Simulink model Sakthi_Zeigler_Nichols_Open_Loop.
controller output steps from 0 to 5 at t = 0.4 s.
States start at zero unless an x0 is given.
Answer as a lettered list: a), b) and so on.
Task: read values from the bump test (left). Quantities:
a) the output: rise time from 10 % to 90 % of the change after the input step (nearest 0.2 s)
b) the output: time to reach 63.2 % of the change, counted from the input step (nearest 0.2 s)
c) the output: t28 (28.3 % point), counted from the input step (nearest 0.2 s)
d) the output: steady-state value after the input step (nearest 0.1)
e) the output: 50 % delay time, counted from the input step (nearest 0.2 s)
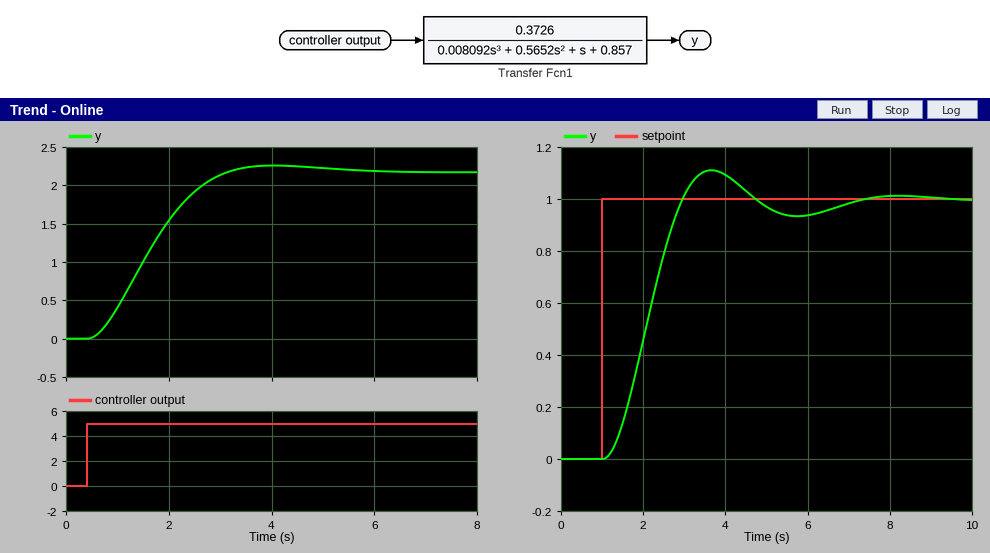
a) 1.8 s
b) 1.4 s
c) 0.8 s
d) 2.2
e) 1.2 s
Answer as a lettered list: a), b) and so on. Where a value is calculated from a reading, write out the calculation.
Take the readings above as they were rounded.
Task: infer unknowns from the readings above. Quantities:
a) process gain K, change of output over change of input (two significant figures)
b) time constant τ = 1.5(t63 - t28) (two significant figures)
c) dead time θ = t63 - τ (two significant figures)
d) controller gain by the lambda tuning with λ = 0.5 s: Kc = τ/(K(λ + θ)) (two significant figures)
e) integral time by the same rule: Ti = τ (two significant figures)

a) (2.2 - 0) / 5 = 0.44
b) 1.5 × (1.4 - 0.8) = 0.90 s
c) 1.4 - 0.9 = 0.50 s
d) 0.9 / (0.44 × (0.5 + 0.5)) = 2.0
e) 0.90 s
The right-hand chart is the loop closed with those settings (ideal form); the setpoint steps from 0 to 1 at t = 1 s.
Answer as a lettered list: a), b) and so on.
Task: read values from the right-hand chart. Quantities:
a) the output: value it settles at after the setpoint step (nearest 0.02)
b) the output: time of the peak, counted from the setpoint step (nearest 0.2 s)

a) 1.00
b) 2.6 s
